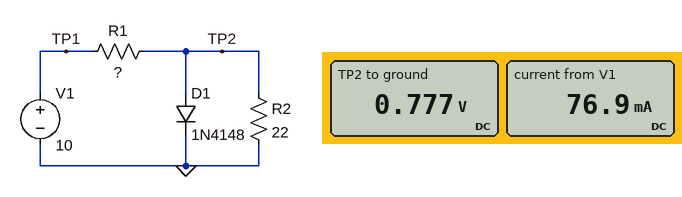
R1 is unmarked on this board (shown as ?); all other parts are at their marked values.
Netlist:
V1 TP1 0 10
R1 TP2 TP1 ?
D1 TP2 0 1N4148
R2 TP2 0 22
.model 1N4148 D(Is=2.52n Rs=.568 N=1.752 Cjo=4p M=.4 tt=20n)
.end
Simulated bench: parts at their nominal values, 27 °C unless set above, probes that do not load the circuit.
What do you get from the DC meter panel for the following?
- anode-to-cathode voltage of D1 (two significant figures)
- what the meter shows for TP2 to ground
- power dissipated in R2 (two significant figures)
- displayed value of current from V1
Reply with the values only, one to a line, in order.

780 mV
0.777 V
27 mW
76.9 mA
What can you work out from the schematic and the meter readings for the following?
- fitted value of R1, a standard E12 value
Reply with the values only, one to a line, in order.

120 Ω
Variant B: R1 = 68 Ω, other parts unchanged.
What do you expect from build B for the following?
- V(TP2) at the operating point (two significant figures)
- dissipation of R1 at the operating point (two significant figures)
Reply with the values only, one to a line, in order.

850 mV
1.2 W
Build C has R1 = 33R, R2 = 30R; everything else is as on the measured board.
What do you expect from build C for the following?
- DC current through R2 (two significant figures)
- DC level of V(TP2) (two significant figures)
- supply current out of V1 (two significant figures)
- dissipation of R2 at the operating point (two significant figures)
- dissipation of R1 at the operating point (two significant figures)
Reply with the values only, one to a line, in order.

32 mA
970 mV
270 mA
31 mW
2.5 W
